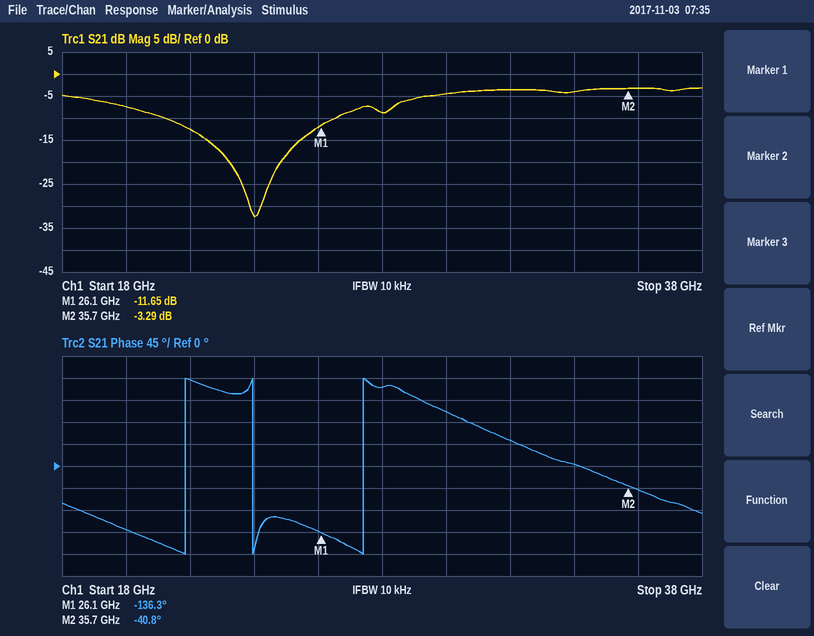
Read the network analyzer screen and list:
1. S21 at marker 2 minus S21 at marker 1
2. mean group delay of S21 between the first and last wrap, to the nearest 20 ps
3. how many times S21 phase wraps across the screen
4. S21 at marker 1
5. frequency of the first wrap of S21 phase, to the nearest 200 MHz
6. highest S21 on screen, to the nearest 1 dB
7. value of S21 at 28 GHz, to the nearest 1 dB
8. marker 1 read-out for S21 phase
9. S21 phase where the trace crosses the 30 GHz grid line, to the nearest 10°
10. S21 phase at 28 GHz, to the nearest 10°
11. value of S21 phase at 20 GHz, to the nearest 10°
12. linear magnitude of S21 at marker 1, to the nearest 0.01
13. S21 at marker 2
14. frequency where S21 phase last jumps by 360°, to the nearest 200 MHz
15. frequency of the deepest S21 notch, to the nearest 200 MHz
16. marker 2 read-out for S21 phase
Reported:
8.36 dB
360 ps
3
-11.65 dB
21.8 GHz
-3 dB
-9 dB
-136.3°
110°
160°
-130°
0.26
-3.29 dB
27.4 GHz
24.0 GHz
-40.8°
